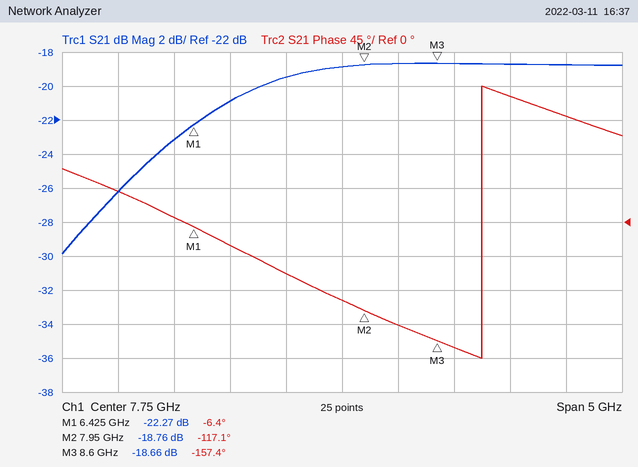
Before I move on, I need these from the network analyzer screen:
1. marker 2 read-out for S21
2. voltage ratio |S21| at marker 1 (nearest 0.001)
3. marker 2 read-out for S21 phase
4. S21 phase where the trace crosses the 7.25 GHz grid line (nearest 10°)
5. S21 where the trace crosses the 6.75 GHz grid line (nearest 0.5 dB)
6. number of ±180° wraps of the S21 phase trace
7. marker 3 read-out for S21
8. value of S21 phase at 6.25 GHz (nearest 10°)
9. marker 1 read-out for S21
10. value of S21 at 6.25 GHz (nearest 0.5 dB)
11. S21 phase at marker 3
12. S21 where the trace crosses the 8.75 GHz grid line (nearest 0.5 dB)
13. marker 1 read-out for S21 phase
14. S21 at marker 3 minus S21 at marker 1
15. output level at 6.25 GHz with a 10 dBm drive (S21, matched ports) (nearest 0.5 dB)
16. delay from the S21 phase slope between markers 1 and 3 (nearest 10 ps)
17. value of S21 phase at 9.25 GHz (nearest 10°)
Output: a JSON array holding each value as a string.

["-18.76 dB", "0.077", "-117.1°", "-70°", "-21.0 dB", "1", "-18.66 dB", "10°", "-22.27 dB", "-23.0 dB", "-157.4°", "-18.5 dB", "-6.4°", "3.61 dB", "-13.0 dBm", "190 ps", "170°"]
